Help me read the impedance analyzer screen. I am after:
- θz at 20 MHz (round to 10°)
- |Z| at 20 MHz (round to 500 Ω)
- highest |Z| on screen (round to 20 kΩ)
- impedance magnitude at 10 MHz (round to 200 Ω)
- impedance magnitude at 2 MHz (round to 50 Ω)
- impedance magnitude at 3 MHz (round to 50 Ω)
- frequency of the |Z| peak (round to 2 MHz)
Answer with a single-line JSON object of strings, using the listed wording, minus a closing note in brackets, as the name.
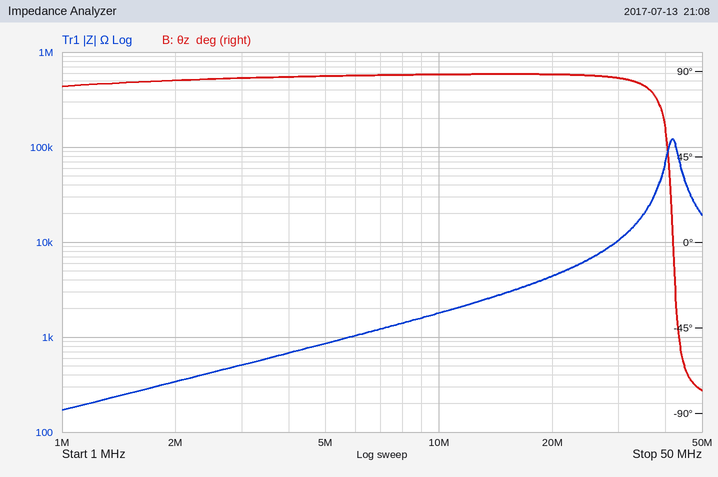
{"θz at 20 MHz": "90°", "|Z| at 20 MHz": "4.5 kΩ", "highest |Z| on screen": "120 kΩ", "impedance magnitude at 10 MHz": "1.8 kΩ", "impedance magnitude at 2 MHz": "350 Ω", "impedance magnitude at 3 MHz": "500 Ω", "frequency of the |Z| peak": "42 MHz"}
